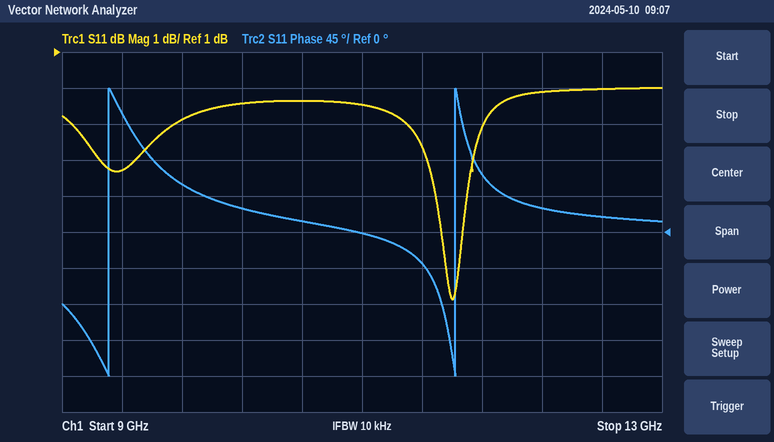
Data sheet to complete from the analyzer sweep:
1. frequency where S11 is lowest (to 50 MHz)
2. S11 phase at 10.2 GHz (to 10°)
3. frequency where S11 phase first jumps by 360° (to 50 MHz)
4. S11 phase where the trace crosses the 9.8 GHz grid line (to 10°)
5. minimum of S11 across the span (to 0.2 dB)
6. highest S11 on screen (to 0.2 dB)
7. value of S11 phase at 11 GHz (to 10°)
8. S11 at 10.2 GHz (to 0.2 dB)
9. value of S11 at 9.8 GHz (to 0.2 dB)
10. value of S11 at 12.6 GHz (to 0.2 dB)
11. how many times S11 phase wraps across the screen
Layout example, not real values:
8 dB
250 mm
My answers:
11.60 GHz
30°
9.30 GHz
60°
-5.8 dB
0.0 dB
0°
-0.4 dB
-0.8 dB
0.0 dB
2
